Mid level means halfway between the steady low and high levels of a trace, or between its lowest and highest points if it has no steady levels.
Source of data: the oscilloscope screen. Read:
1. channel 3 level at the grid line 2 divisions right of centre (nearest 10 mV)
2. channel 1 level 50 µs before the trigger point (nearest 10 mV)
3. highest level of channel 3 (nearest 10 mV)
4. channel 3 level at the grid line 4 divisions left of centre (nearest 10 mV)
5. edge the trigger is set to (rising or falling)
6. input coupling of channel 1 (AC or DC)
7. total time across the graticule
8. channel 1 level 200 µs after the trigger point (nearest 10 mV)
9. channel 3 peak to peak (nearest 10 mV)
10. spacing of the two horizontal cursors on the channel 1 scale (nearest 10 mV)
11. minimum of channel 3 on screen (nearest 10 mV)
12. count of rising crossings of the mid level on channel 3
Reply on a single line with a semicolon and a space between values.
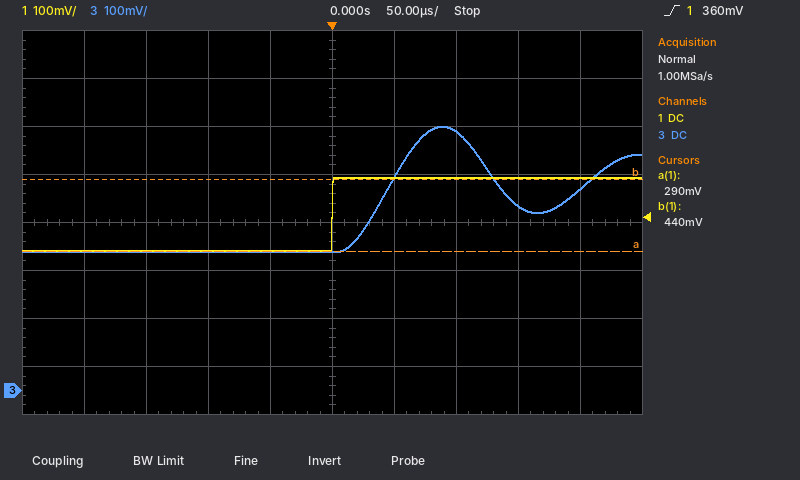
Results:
540 mV; 290 mV; 550 mV; 290 mV; rising; DC; 500 µs; 440 mV; 260 mV; 150 mV; 290 mV; 2
